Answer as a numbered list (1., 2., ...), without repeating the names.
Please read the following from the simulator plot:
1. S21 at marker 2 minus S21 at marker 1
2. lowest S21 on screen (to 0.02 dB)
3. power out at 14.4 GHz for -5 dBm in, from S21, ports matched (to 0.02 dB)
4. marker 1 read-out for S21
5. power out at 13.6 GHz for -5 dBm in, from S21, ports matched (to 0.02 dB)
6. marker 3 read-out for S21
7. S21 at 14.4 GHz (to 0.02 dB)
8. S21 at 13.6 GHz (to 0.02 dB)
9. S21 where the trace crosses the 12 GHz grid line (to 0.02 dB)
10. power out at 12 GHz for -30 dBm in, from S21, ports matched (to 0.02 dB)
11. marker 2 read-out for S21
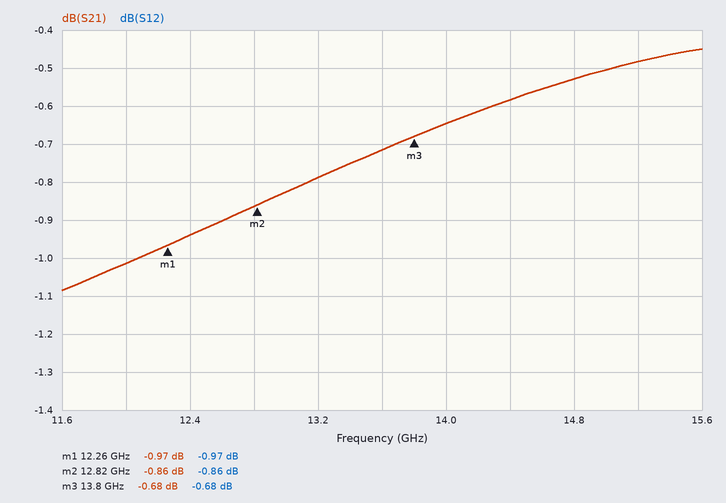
1. 0.11 dB
2. -1.08 dB
3. -5.58 dBm
4. -0.97 dB
5. -5.72 dBm
6. -0.68 dB
7. -0.58 dB
8. -0.72 dB
9. -1.02 dB
10. -31.02 dBm
11. -0.86 dB
